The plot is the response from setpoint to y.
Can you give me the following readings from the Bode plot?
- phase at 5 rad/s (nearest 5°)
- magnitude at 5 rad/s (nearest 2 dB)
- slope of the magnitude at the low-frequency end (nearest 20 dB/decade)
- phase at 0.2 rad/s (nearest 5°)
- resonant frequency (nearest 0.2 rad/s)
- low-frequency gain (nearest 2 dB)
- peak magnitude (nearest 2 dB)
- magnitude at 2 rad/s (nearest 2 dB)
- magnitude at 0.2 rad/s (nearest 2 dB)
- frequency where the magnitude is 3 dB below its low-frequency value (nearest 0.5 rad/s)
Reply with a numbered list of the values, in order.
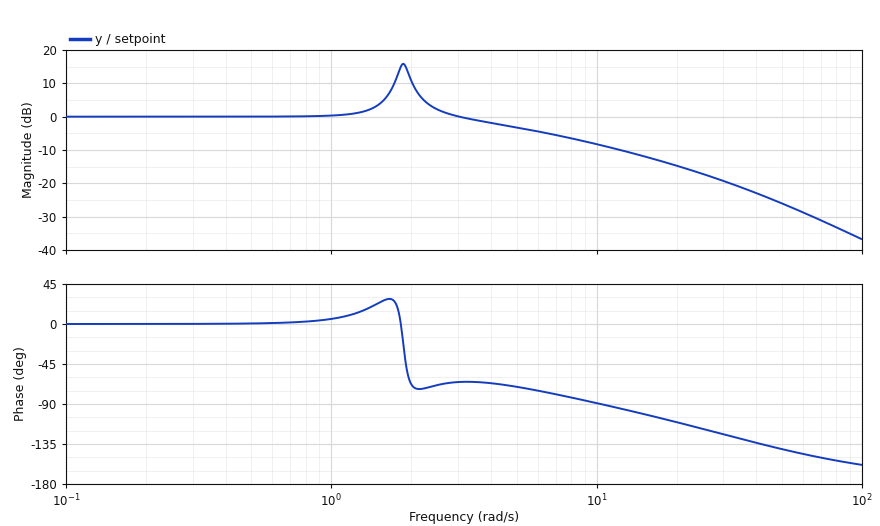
1. -70°
2. -4 dB
3. 0 dB/decade
4. 0°
5. 1.8 rad/s
6. 0 dB
7. 16 dB
8. 10 dB
9. 0 dB
10. 5.0 rad/s
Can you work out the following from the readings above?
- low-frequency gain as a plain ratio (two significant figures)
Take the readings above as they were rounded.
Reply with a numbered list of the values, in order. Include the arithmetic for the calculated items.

1. 10^(0 / 20) = 1.0
